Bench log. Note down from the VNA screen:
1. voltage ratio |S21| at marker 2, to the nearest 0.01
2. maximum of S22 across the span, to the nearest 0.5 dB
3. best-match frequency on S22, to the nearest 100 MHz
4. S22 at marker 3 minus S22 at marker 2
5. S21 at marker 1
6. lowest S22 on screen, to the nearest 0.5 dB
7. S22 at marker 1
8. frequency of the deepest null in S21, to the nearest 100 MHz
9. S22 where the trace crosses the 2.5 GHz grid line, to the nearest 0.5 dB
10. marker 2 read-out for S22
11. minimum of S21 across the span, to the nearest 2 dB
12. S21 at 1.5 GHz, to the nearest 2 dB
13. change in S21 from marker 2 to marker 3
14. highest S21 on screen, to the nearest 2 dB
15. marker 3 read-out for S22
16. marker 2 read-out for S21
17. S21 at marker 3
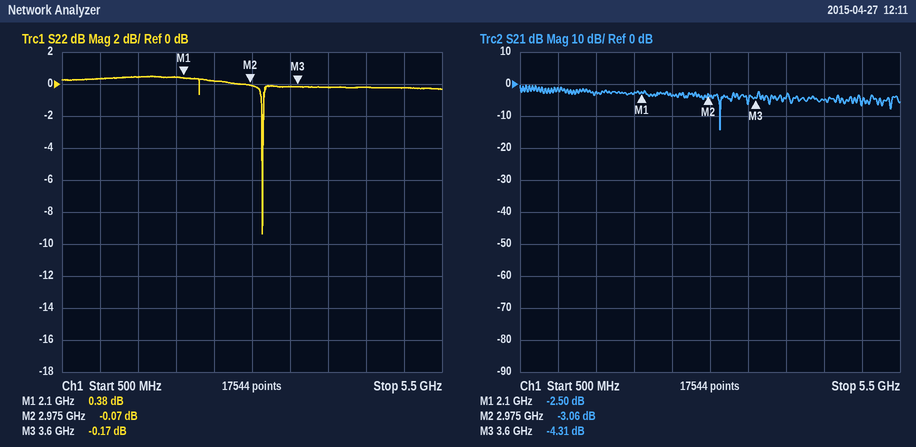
0.70
0.5 dB
3.1 GHz
-0.10 dB
-2.50 dB
-9.5 dB
0.38 dB
3.1 GHz
0.0 dB
-0.07 dB
-14 dB
-2 dB
-1.25 dB
0 dB
-0.17 dB
-3.06 dB
-4.31 dB
